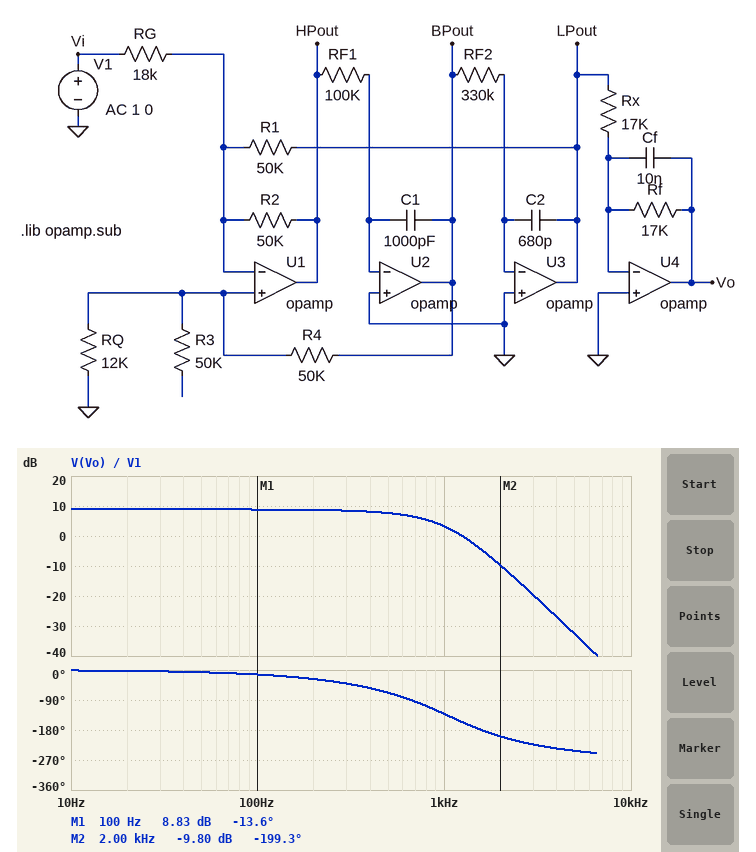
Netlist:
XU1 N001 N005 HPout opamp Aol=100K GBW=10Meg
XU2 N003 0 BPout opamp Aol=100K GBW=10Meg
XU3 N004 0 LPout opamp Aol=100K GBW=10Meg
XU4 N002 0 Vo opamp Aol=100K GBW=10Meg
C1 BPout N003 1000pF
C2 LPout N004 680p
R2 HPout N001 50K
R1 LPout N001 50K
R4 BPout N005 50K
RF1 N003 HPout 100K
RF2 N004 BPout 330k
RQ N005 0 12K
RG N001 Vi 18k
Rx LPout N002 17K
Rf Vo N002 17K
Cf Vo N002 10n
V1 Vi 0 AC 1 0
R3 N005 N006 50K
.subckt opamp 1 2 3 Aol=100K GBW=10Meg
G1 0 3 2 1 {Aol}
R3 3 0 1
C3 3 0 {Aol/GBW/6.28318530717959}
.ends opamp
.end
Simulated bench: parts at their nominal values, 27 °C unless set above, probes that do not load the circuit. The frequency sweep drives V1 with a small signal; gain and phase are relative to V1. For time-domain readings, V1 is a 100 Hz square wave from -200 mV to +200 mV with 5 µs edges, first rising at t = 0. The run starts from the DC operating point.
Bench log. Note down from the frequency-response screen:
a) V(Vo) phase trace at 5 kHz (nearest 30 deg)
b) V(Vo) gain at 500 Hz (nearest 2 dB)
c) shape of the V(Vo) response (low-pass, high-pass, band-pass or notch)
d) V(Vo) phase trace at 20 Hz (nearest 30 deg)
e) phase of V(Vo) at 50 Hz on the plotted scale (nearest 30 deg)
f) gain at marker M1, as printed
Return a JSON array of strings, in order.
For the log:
["-240 deg", "8 dB", "low-pass", "0 deg", "0 deg", "8.83 dB"]
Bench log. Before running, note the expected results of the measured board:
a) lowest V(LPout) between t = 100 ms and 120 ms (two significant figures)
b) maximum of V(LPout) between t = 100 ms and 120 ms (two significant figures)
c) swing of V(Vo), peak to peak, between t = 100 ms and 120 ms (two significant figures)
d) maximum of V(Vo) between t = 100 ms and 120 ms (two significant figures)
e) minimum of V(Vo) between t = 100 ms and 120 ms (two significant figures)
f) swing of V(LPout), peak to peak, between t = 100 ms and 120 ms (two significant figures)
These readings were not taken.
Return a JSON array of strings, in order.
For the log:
["-610 mV", "610 mV", "1.1 V", "570 mV", "-570 mV", "1.2 V"]
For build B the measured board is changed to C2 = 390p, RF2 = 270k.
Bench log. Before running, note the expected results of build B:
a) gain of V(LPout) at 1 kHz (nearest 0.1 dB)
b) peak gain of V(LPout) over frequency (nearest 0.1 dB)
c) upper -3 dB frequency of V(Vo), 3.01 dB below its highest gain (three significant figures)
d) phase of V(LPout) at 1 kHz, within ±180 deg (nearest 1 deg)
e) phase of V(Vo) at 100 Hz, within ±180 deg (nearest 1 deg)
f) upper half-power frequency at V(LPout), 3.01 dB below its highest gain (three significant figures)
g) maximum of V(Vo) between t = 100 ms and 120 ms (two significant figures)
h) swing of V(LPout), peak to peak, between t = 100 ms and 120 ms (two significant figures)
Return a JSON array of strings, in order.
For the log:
["10.3 dB", "10.4 dB", "1.26 kHz", "134 deg", "-10 deg", "1.83 kHz", "570 mV", "1.5 V"]
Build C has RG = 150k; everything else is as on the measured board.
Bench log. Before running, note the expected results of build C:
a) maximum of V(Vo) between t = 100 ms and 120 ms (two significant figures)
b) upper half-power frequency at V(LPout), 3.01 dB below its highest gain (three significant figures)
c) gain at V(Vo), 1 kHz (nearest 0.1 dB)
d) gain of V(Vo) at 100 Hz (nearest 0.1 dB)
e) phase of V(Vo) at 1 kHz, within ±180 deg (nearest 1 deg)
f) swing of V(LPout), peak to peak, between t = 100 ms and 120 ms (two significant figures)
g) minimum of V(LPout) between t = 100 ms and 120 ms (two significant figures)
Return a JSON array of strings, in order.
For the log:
["89 mV", "1.26 kHz", "-9.1 dB", "-9.5 dB", "-127 deg", "220 mV", "-110 mV"]
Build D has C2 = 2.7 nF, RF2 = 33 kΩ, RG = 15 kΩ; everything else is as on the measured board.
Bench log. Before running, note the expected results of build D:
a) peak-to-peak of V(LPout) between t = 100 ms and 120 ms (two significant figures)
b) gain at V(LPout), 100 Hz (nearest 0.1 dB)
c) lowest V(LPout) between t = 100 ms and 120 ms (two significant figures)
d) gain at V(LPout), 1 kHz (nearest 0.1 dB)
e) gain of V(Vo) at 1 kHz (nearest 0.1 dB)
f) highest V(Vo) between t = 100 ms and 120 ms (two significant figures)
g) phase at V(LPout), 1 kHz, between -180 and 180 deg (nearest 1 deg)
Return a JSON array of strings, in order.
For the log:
["1.8 V", "10.5 dB", "-900 mV", "11.7 dB", "8.4 dB", "670 mV", "138 deg"]
